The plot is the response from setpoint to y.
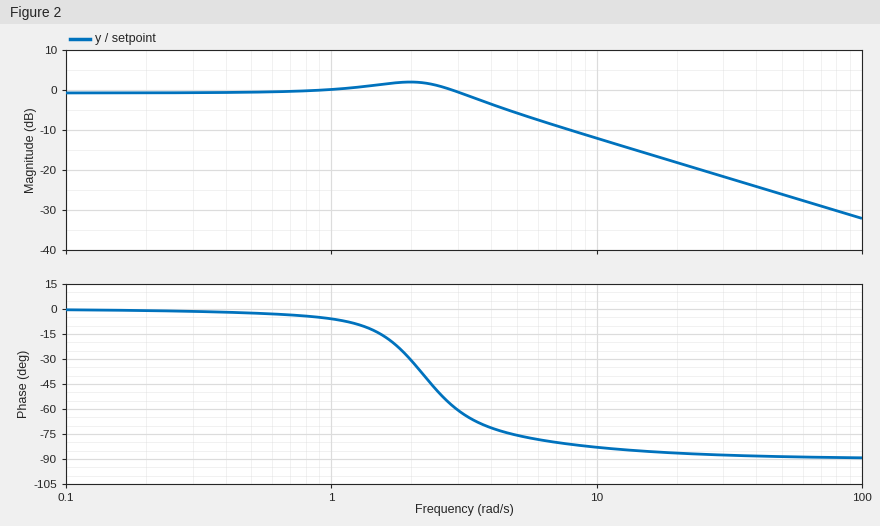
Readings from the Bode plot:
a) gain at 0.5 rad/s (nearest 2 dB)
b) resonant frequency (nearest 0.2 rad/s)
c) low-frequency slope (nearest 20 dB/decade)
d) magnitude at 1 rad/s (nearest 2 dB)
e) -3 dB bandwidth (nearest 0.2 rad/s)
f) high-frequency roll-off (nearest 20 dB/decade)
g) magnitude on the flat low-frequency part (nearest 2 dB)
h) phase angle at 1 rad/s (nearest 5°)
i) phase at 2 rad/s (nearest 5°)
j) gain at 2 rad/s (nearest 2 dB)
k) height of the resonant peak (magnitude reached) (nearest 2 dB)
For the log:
0 dB
2.0 rad/s
0 dB/decade
0 dB
4.0 rad/s
-20 dB/decade
0 dB
-5°
-30°
2 dB
2 dB
